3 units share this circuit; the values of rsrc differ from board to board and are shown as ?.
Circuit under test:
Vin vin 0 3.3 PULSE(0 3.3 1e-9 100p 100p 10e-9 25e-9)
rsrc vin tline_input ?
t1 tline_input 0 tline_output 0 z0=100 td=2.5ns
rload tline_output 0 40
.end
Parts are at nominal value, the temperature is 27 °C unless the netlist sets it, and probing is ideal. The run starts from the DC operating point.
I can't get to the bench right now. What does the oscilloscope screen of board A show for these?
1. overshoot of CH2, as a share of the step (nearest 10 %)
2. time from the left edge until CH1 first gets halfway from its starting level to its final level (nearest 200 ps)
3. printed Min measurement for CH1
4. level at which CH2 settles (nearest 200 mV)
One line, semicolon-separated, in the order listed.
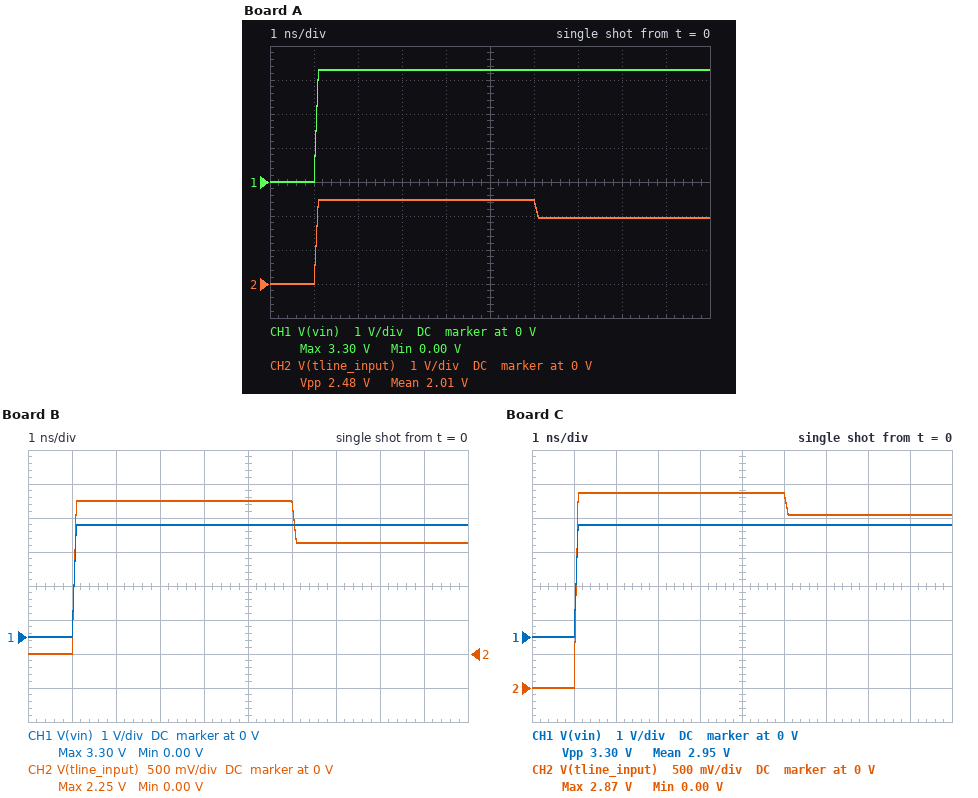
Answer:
30 %; 1.0 ns; 0.00 V; 2.0 V
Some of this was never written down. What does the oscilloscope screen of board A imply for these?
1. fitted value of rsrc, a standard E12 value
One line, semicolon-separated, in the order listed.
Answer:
33 Ω
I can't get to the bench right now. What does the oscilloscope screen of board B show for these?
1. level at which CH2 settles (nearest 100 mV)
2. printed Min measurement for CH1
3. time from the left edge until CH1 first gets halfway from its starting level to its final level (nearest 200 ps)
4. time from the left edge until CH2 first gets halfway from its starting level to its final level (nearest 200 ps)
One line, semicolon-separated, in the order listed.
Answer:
1.6 V; 0.00 V; 1.0 ns; 1.0 ns
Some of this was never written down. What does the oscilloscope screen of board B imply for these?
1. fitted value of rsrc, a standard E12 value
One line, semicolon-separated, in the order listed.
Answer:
47 Ω
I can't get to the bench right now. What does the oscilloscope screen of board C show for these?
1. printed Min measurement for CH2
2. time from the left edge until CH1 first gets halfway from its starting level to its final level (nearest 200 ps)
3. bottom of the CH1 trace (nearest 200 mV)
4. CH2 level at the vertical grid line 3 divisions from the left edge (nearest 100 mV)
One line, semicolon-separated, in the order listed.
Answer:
0.00 V; 1.0 ns; 0 V; 2.9 V
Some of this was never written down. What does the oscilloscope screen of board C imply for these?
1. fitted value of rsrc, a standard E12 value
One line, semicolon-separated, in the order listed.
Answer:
15 Ω
